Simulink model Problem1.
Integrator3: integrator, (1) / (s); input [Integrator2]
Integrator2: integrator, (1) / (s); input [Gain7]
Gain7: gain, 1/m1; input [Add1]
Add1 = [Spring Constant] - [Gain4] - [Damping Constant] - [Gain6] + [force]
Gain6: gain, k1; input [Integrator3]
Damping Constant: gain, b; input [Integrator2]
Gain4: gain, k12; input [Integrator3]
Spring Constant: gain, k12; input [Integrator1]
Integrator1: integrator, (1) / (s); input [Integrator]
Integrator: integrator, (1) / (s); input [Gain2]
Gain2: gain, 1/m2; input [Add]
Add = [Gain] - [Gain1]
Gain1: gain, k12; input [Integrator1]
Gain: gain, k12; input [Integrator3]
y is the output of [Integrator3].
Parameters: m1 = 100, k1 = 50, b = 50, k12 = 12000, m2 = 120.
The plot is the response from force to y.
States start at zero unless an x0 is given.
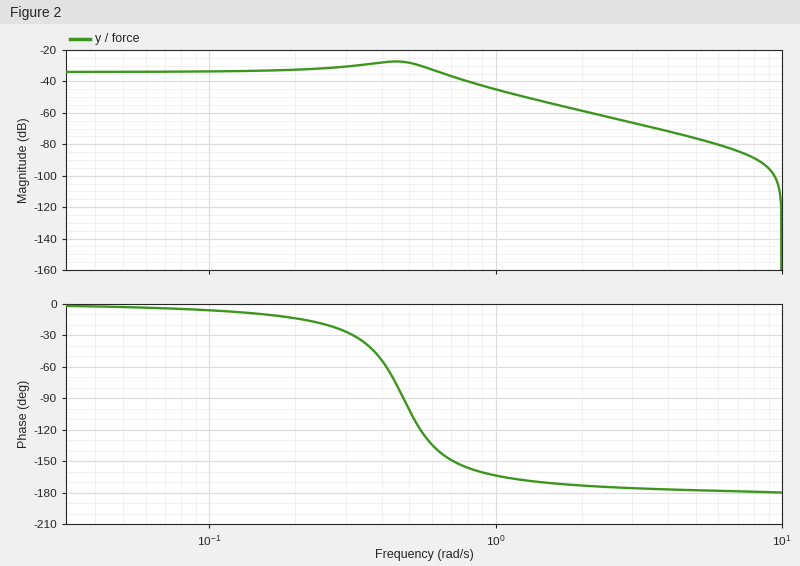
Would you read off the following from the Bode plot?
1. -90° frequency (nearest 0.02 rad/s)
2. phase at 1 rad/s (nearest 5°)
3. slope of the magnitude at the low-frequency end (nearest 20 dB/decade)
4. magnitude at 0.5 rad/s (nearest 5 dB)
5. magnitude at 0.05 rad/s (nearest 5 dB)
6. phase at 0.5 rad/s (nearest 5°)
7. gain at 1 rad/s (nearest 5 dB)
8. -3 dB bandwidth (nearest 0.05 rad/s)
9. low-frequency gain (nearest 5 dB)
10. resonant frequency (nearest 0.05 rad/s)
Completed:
0.48 rad/s
-165°
0 dB/decade
-30 dB
-35 dB
-100°
-45 dB
0.70 rad/s
-35 dB
0.45 rad/s
